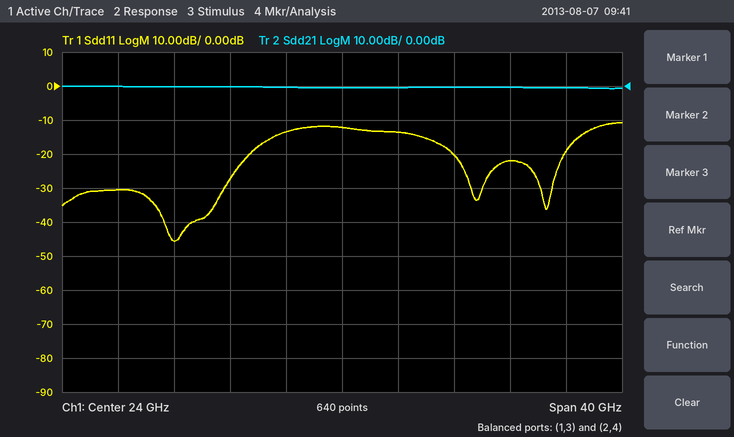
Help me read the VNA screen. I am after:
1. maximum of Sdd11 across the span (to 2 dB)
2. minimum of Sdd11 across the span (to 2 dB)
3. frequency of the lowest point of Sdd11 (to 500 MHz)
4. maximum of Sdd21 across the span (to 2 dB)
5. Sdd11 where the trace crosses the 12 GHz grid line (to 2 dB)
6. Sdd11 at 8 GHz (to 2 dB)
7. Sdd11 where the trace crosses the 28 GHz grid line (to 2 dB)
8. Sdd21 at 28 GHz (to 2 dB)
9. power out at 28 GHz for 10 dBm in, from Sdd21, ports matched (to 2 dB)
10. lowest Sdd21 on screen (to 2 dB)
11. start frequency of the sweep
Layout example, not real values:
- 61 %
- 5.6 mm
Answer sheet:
- -10 dB
- -46 dB
- 12.0 GHz
- 0 dB
- -46 dB
- -30 dB
- -14 dB
- 0 dB
- 10 dBm
- 0 dB
- 4 GHz
